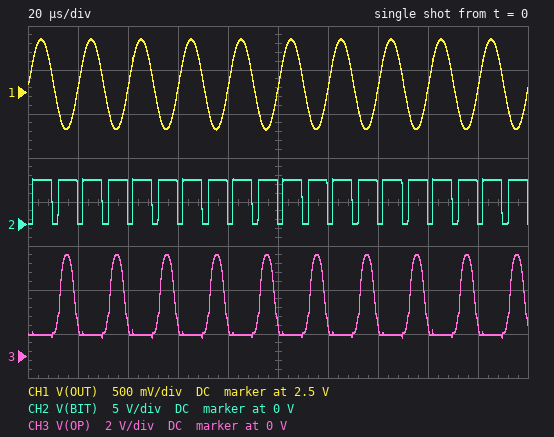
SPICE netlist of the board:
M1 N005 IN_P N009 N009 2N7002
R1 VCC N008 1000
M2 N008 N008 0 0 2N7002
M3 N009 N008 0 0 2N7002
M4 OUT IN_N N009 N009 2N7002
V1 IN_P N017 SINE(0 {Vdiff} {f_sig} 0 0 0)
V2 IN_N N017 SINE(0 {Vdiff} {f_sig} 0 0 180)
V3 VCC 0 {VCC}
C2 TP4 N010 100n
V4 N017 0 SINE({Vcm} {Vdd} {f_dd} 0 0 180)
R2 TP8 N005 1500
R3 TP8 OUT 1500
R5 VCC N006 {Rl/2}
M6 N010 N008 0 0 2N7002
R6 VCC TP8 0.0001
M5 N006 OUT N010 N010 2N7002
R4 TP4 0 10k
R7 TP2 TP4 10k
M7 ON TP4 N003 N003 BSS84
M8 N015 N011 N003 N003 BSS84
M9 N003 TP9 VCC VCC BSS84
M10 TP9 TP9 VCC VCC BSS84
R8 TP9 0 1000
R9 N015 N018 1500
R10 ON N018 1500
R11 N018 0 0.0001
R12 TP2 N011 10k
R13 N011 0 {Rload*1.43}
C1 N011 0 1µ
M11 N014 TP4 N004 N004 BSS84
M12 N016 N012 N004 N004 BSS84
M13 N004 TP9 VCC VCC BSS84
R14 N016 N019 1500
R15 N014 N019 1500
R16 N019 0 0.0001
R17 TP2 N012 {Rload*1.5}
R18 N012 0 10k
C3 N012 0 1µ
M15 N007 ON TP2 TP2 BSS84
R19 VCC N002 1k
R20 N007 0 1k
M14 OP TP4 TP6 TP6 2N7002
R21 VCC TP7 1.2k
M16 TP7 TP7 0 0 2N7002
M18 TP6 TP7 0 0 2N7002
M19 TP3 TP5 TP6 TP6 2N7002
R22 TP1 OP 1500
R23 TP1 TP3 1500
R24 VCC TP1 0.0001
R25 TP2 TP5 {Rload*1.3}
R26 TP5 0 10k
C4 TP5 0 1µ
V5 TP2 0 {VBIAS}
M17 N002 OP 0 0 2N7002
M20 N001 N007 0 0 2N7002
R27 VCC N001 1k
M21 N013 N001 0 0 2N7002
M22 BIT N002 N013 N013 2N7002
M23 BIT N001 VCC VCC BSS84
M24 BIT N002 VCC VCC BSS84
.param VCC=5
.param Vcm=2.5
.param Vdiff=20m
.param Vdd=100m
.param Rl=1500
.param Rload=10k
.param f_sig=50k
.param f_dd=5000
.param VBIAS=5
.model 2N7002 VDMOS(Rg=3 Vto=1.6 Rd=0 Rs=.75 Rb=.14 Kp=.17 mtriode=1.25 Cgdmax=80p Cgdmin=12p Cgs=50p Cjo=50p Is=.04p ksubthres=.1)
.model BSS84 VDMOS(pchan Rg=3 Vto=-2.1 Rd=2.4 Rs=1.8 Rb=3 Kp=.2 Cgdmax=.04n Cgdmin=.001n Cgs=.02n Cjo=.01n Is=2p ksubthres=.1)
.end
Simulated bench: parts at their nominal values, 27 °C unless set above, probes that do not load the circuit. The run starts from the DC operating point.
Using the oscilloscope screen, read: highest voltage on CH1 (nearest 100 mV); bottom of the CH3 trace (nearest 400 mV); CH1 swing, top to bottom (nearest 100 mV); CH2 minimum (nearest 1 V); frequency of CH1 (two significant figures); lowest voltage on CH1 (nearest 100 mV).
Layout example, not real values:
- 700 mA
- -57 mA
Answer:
- 3.1 V
- 800 mV
- 1.0 V
- 0 V
- 50 kHz
- 2.1 V
